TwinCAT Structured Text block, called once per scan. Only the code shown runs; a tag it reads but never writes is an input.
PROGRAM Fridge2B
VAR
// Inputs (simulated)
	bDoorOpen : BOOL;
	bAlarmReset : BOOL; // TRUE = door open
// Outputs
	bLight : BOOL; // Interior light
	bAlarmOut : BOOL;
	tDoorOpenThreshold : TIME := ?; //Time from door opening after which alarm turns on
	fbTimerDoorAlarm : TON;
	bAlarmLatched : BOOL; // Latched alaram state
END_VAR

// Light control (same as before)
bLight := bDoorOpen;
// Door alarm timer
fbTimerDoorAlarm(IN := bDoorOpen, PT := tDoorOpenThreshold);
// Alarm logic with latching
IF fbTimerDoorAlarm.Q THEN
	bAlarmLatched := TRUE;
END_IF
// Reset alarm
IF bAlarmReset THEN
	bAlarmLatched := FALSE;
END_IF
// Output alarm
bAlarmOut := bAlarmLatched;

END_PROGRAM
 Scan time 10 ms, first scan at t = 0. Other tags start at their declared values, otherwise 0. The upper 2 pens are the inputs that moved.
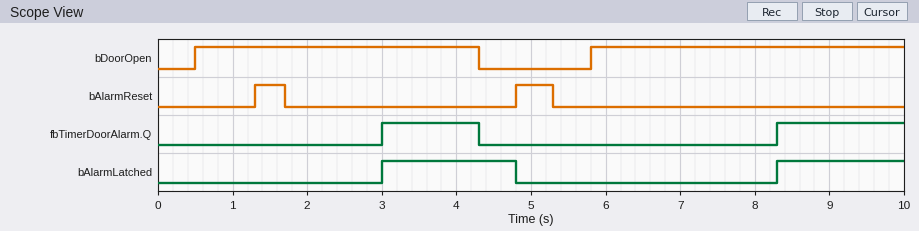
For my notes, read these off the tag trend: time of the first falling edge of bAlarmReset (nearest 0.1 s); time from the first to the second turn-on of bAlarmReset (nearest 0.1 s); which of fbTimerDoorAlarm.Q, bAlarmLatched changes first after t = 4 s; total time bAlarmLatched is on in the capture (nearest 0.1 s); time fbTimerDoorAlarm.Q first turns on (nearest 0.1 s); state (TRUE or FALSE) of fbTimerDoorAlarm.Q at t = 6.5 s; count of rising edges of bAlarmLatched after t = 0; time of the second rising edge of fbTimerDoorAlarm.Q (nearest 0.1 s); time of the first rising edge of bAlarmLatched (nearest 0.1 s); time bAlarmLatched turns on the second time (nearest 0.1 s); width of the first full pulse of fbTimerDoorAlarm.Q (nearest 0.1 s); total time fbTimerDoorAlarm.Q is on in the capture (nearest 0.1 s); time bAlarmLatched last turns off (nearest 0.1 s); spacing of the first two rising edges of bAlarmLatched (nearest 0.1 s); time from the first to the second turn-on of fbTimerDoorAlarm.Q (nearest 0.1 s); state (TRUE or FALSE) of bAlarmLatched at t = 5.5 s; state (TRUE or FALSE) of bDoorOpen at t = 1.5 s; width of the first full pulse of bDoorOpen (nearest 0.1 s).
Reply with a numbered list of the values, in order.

1. 1.7 s
2. 3.5 s
3. fbTimerDoorAlarm.Q
4. 3.5 s
5. 3.0 s
6. FALSE
7. 2
8. 8.3 s
9. 3.0 s
10. 8.3 s
11. 1.3 s
12. 3.0 s
13. 4.8 s
14. 5.3 s
15. 5.3 s
16. FALSE
17. TRUE
18. 3.8 s
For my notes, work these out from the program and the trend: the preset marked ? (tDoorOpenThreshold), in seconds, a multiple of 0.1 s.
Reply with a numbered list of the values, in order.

1. 2.5 s
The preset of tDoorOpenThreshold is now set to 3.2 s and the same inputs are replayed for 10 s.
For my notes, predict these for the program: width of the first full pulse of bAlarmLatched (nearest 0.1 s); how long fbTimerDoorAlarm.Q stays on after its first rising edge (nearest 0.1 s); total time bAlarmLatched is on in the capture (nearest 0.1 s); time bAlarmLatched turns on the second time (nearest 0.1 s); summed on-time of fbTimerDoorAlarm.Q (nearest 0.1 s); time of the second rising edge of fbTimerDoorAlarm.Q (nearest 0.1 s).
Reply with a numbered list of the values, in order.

1. 1.1 s
2. 0.6 s
3. 2.1 s
4. 9.0 s
5. 1.6 s
6. 9.0 s
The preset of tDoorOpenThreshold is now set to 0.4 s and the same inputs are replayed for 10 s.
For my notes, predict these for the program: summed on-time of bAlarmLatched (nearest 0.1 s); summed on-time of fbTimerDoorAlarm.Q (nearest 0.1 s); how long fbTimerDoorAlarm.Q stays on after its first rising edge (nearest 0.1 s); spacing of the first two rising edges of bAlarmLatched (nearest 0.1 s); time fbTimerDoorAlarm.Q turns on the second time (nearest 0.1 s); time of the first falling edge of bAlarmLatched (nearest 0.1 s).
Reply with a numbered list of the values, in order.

1. 7.3 s
2. 7.2 s
3. 3.4 s
4. 0.8 s
5. 6.2 s
6. 1.3 s
